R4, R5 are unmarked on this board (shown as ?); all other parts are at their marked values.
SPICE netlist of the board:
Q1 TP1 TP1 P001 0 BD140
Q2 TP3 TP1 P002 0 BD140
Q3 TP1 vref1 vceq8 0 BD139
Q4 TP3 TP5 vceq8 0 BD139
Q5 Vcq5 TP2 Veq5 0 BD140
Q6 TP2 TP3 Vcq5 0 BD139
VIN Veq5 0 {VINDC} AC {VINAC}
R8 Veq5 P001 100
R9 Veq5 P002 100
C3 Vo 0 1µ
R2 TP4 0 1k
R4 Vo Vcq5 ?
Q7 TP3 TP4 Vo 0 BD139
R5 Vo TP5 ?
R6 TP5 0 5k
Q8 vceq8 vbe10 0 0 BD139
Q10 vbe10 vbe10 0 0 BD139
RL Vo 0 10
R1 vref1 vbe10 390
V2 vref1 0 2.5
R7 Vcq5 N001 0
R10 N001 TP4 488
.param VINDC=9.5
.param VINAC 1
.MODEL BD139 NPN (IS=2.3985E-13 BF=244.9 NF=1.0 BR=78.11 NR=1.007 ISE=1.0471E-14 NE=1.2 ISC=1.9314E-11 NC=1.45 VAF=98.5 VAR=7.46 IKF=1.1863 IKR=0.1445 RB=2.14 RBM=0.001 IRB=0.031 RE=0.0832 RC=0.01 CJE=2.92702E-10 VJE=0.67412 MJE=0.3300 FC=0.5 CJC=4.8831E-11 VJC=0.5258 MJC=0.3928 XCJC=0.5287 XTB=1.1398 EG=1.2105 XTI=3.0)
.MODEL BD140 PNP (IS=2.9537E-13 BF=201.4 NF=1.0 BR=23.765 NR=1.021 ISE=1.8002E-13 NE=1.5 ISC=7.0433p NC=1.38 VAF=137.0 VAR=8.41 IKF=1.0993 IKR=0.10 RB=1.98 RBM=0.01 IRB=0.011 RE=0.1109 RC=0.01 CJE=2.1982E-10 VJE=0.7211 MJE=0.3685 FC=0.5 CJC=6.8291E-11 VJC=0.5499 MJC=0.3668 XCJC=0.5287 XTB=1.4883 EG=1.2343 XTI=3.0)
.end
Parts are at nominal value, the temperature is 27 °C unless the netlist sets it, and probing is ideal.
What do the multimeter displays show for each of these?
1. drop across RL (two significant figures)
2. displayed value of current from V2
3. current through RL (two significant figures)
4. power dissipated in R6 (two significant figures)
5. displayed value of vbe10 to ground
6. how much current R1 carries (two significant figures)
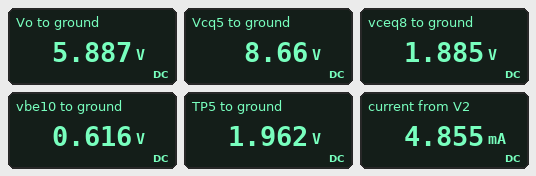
5.9 V
4.855 mA
590 mA
770 µW
0.616 V
4.8 mA
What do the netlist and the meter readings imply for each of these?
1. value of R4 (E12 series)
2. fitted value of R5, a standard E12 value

4.7 Ω
10 kΩ
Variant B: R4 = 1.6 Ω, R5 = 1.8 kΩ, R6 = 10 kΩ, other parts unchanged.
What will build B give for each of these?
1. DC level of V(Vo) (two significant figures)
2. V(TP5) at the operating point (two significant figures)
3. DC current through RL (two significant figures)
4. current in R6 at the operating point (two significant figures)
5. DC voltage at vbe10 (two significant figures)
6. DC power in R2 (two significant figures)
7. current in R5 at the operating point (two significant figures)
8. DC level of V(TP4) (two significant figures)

3.0 V
2.5 V
300 mA
250 µA
620 mV
5.4 mW
260 µA
2.3 V
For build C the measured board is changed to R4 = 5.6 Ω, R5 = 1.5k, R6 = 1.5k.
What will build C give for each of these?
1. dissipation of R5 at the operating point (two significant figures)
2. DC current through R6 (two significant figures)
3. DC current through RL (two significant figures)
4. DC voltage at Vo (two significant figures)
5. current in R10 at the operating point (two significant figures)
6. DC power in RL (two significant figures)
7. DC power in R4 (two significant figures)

4.2 mW
1.7 mA
500 mA
5.0 V
5.3 mA
2.5 W
1.4 W
